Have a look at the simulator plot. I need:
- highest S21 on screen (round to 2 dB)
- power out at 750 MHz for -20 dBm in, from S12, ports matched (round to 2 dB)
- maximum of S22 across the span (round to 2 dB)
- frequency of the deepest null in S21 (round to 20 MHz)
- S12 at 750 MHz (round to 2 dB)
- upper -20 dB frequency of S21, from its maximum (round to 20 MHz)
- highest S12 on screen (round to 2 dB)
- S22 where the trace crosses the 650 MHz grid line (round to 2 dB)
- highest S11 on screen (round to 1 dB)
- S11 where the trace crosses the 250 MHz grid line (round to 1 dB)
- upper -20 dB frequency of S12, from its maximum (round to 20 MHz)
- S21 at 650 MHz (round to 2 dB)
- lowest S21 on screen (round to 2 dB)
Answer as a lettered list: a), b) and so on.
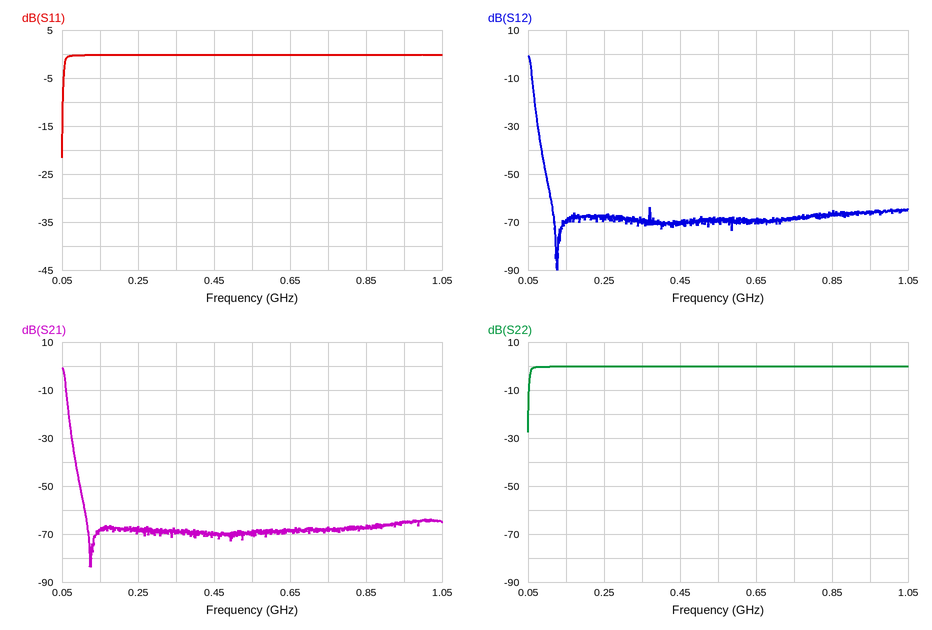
a) 0 dB
b) -88 dBm
c) 0 dB
d) 120 MHz
e) -68 dB
f) 60 MHz
g) 0 dB
h) 0 dB
i) 0 dB
j) 0 dB
k) 60 MHz
l) -68 dB
m) -84 dB
